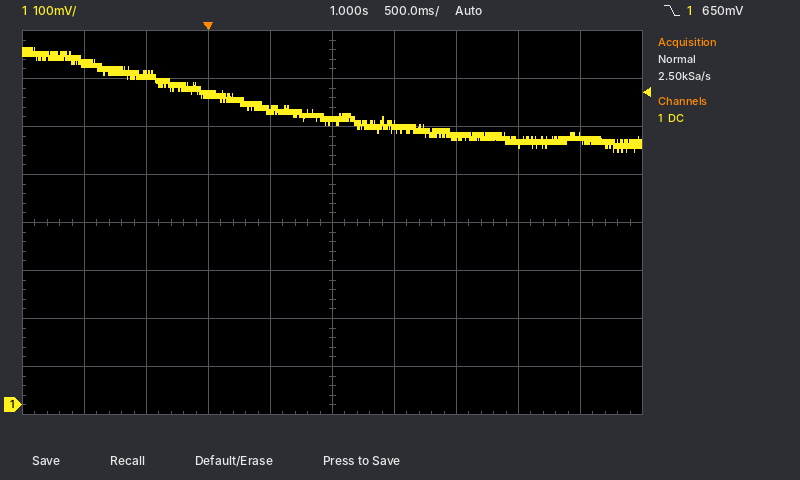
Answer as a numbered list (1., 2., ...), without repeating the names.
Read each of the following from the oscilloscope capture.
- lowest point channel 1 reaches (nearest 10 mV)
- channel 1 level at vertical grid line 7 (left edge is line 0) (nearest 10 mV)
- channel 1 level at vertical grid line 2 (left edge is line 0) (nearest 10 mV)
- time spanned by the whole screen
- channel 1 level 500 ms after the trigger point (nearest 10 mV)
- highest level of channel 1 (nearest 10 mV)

1. 530 mV
2. 560 mV
3. 690 mV
4. 5 s
5. 620 mV
6. 740 mV
